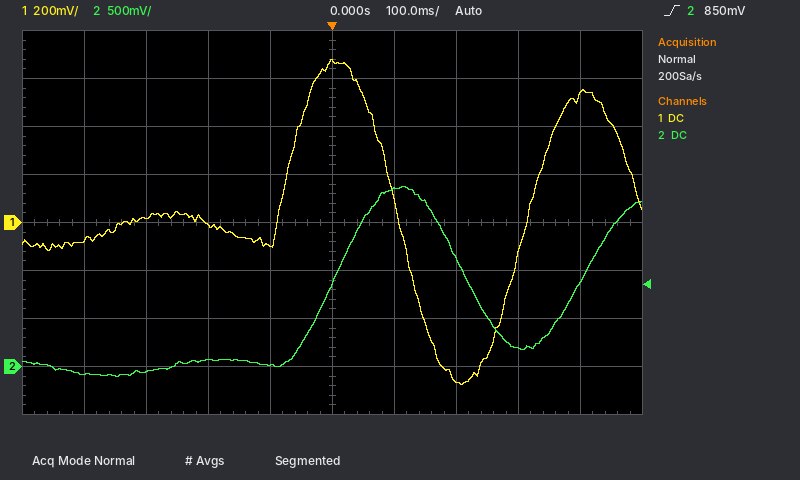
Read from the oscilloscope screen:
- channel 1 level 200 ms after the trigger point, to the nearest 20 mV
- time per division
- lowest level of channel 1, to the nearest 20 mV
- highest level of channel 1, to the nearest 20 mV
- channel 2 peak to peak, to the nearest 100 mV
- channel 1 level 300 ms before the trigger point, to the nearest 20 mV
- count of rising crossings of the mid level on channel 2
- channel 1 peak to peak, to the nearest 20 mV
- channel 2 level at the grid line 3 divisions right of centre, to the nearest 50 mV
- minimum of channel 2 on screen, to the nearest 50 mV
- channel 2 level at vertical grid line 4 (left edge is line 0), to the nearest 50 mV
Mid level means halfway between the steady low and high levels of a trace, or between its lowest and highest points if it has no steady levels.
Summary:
-660 mV
100 ms
-680 mV
680 mV
2.00 V
20 mV
2
1.36 V
200 mV
-100 mV
0 mV
